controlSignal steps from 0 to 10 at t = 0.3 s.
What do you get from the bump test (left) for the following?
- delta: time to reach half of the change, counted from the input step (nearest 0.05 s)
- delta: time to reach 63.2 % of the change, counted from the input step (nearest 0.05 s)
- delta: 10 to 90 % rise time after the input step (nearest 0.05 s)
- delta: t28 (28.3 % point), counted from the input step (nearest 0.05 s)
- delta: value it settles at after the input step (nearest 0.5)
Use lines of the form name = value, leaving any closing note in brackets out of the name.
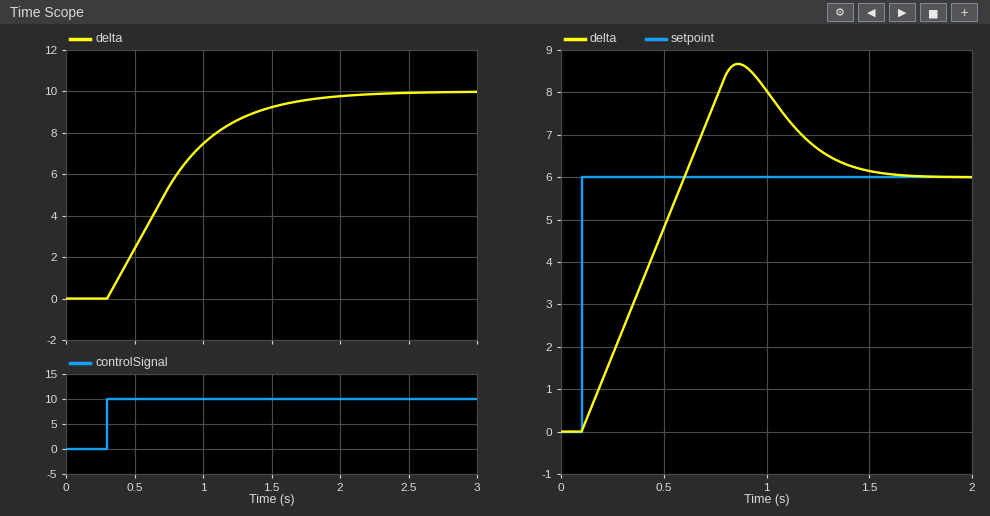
delta: time to reach half of the change, counted from the input step = 0.40 s
delta: time to reach 63.2 % of the change, counted from the input step = 0.55 s
delta: 10 to 90 % rise time after the input step = 1.00 s
delta: t28 (28.3 % point), counted from the input step = 0.25 s
delta: value it settles at after the input step = 10.0
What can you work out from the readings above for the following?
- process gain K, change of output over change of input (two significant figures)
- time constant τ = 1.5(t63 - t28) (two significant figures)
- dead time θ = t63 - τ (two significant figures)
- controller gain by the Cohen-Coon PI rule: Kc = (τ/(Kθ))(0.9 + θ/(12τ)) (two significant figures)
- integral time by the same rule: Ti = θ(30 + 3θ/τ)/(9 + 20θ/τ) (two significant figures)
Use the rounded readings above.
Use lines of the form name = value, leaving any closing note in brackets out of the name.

process gain K, change of output over change of input = 1.0
time constant τ = 1.5(t63 - t28) = 0.45 s
dead time θ = t63 - τ = 0.10 s
controller gain by the Cohen-Coon PI rule: Kc = (τ/(Kθ))(0.9 + θ/(12τ)) = 4.1
integral time by the same rule: Ti = θ(30 + 3θ/τ)/(9 + 20θ/τ) = 0.23 s
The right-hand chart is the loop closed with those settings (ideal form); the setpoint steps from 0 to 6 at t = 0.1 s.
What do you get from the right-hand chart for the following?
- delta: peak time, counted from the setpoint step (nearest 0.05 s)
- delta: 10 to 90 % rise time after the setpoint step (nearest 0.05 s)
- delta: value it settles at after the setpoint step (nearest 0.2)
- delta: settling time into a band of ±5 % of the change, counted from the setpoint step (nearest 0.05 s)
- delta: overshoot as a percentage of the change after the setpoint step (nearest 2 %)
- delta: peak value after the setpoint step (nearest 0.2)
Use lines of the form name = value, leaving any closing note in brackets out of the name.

delta: peak time, counted from the setpoint step = 0.75 s
delta: 10 to 90 % rise time after the setpoint step = 0.40 s
delta: value it settles at after the setpoint step = 6.0
delta: settling time into a band of ±5 % of the change, counted from the setpoint step = 1.30 s
delta: overshoot as a percentage of the change after the setpoint step = 44 %
delta: peak value after the setpoint step = 8.6
